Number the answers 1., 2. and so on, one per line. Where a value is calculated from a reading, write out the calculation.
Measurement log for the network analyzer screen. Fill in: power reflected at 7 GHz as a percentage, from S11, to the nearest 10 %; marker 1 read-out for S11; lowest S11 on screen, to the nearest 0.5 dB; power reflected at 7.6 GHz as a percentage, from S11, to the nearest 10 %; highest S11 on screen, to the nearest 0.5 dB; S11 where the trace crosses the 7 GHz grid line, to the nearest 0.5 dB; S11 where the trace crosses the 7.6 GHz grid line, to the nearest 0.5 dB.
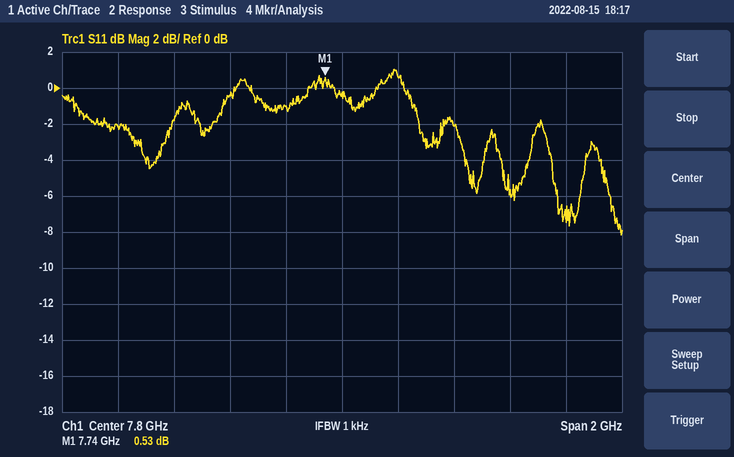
1. 10^(-2/10) ≈ 63.1 %, so 60 % to the nearest 10 %
2. 0.53 dB
3. -8.0 dB
4. 10^(-1/10) ≈ 79.4 %, so 80 % to the nearest 10 %
5. 1.0 dB
6. -2.0 dB
7. -1.0 dB
